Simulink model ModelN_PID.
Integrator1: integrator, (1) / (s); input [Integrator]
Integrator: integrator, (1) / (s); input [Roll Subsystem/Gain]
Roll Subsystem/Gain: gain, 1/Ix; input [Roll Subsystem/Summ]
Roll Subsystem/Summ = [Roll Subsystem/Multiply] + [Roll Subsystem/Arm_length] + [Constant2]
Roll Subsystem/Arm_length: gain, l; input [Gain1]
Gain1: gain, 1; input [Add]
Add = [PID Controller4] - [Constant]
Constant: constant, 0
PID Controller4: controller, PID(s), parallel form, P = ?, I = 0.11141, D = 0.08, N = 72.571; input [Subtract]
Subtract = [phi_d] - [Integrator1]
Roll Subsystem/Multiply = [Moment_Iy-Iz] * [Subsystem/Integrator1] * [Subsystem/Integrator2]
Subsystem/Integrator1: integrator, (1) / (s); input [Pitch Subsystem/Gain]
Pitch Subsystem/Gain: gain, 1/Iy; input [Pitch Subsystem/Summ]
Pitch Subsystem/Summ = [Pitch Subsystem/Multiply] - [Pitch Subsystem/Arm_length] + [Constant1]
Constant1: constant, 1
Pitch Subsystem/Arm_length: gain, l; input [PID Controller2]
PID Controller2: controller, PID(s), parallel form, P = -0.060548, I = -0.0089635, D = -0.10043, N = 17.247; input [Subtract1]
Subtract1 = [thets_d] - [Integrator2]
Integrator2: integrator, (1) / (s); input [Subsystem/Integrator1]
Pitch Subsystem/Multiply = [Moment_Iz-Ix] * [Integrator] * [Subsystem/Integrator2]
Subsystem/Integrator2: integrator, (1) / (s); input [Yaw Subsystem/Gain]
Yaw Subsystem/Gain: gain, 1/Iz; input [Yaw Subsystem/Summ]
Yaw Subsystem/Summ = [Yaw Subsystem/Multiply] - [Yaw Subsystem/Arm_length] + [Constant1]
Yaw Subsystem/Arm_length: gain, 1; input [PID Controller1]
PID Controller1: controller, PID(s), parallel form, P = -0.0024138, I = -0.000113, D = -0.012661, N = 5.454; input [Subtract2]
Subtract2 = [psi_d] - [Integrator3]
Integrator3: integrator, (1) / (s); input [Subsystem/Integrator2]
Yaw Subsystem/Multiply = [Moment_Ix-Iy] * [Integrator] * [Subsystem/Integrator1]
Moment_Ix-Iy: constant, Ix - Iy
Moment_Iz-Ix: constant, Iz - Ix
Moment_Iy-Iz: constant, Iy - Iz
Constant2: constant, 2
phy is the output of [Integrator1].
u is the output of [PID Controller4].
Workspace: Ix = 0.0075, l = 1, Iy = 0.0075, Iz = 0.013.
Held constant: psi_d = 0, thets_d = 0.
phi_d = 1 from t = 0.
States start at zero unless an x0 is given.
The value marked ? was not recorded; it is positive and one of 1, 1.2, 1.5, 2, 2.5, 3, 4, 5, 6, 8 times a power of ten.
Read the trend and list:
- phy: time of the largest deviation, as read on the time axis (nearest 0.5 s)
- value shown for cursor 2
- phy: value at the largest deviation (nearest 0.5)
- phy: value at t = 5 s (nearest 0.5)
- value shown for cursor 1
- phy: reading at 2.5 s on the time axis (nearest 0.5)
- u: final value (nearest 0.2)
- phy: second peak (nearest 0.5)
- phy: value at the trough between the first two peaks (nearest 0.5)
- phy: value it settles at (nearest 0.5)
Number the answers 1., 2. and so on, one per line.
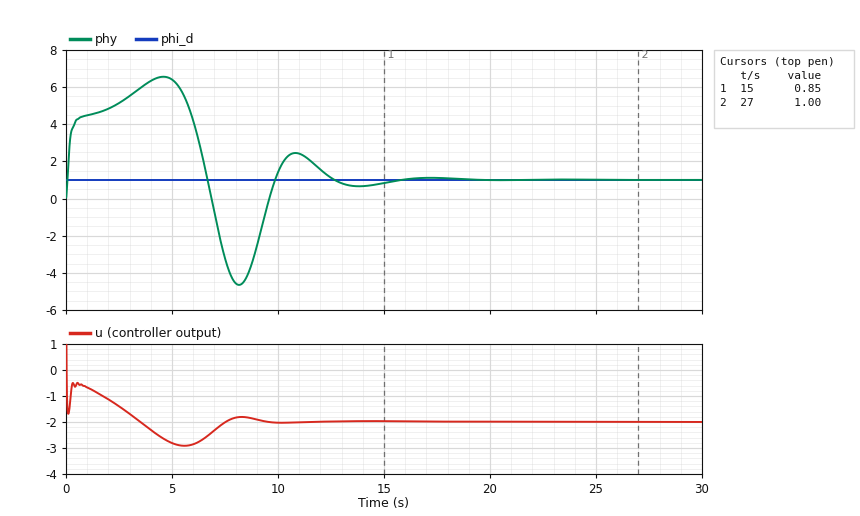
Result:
1. 4.5 s
2. 1.00
3. 6.5
4. 6.5
5. 0.85
6. 5.0
7. -2.0
8. 2.5
9. -4.5
10. 1.0
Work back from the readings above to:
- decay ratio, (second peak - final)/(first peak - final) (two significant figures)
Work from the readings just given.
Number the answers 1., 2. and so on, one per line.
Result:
1. 0.27
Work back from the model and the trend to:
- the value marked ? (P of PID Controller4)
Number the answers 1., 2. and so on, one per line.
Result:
1. 0.1
